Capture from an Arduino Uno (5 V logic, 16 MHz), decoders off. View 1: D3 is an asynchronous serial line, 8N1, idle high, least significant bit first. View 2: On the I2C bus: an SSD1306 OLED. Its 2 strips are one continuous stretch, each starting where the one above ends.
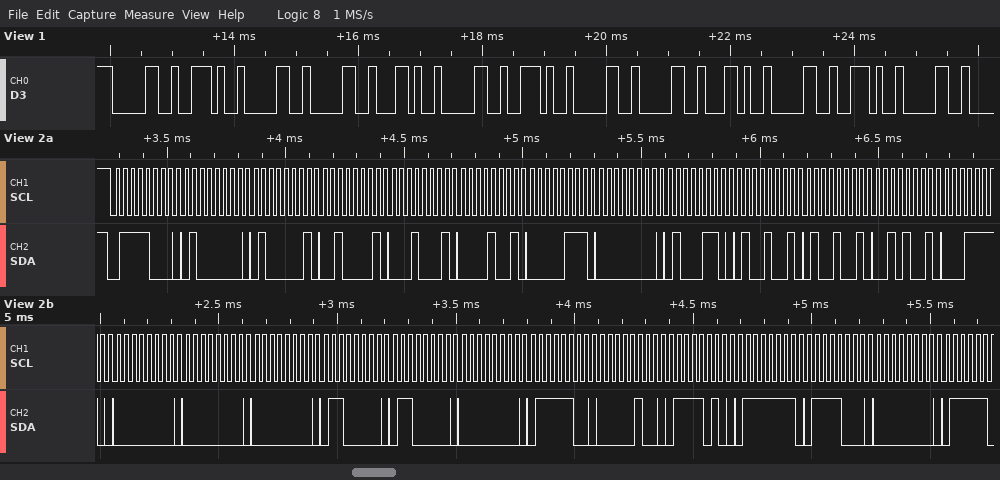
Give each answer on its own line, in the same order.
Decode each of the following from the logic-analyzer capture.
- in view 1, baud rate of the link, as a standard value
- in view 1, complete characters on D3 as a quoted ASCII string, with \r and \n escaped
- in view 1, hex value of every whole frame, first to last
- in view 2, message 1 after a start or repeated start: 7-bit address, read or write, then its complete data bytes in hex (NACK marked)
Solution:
9600 baud
"0.00,0.00,0.0"
30 2E 30 30 2C 30 2E 30 30 2C 30 2E 30
0x3C write: 40 41 21 11 09 07 00 46 49 49 29 1E 00 00 00 60 60 00 7C 04 7A 7F 78 00
